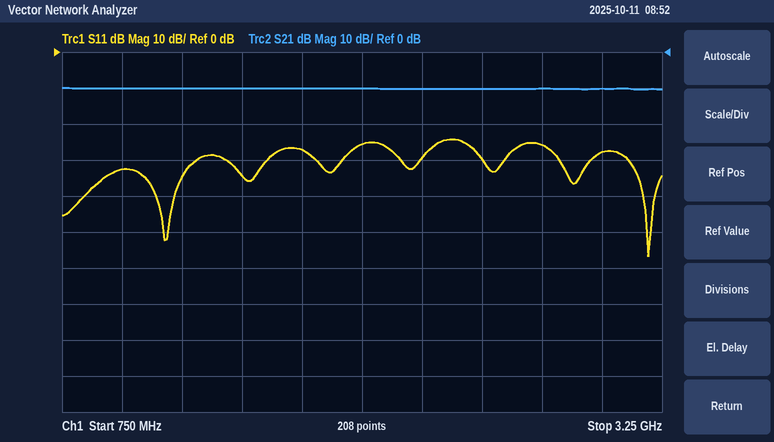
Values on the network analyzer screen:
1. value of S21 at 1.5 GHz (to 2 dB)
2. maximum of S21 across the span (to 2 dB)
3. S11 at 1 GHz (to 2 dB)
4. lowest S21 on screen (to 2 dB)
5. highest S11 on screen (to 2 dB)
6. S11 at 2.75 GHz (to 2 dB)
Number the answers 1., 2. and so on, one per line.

1. -10 dB
2. -10 dB
3. -32 dB
4. -10 dB
5. -24 dB
6. -26 dB
